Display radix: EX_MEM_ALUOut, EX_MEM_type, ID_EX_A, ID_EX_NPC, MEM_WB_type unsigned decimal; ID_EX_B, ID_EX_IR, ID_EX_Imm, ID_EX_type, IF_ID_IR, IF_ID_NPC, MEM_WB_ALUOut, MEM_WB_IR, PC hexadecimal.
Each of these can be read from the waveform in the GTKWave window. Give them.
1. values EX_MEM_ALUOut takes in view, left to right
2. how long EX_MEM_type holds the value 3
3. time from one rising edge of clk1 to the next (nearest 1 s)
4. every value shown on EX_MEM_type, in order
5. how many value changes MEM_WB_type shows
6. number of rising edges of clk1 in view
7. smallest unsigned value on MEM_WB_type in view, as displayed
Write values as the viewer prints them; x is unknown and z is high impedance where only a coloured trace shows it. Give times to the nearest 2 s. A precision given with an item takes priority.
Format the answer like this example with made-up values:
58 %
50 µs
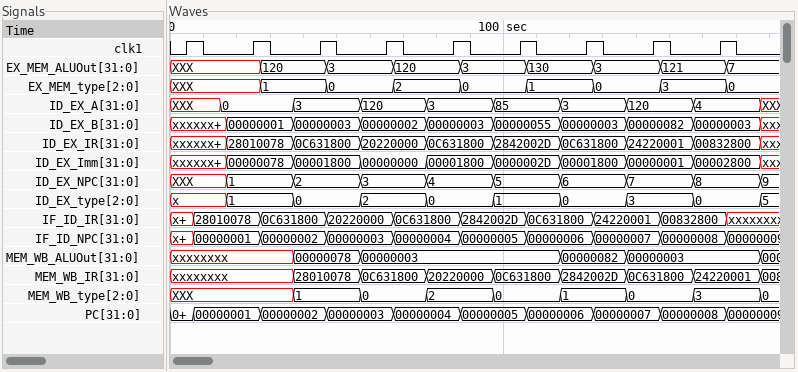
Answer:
XXX, 120, 3, 120, 3, 130, 3, 121, 7
20 s
20 s
XXX, 1, 0, 2, 0, 1, 0, 3, 0
8
9
0
